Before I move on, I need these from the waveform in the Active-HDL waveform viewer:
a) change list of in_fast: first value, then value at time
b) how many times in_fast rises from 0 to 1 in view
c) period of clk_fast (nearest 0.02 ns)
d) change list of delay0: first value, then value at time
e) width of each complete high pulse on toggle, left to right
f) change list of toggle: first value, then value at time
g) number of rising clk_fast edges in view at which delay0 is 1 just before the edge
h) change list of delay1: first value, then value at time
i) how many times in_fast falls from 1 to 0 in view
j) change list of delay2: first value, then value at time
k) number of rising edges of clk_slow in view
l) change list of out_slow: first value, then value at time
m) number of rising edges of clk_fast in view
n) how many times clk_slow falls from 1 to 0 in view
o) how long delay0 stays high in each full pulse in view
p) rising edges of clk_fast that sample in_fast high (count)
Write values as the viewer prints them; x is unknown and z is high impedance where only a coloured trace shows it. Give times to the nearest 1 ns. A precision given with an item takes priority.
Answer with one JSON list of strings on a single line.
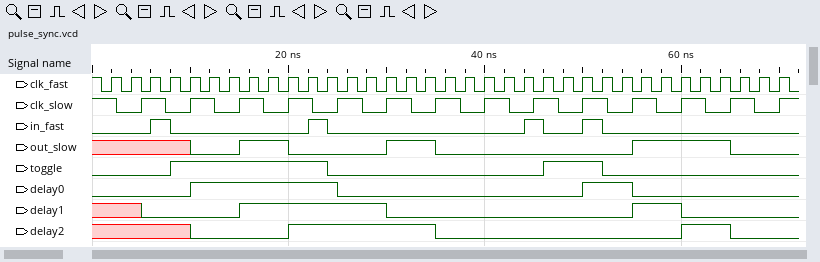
["0, 1 at 6 ns, 0 at 8 ns, 1 at 22 ns, 0 at 24 ns, 1 at 44 ns, 0 at 46 ns, 1 at 50 ns, 0 at 52 ns", "4", "2 ns", "0, 1 at 10 ns, 0 at 25 ns, 1 at 50 ns, 0 at 55 ns", "16 ns, 6 ns", "0, 1 at 8 ns, 0 at 24 ns, 1 at 46 ns, 0 at 52 ns", "9", "x, 0 at 5 ns, 1 at 15 ns, 0 at 30 ns, 1 at 55 ns, 0 at 60 ns", "4", "x, 0 at 10 ns, 1 at 20 ns, 0 at 35 ns, 1 at 60 ns, 0 at 65 ns", "14", "x, 0 at 10 ns, 1 at 15 ns, 0 at 20 ns, 1 at 30 ns, 0 at 35 ns, 1 at 55 ns, 0 at 65 ns", "35", "14", "15 ns, 5 ns", "4"]
